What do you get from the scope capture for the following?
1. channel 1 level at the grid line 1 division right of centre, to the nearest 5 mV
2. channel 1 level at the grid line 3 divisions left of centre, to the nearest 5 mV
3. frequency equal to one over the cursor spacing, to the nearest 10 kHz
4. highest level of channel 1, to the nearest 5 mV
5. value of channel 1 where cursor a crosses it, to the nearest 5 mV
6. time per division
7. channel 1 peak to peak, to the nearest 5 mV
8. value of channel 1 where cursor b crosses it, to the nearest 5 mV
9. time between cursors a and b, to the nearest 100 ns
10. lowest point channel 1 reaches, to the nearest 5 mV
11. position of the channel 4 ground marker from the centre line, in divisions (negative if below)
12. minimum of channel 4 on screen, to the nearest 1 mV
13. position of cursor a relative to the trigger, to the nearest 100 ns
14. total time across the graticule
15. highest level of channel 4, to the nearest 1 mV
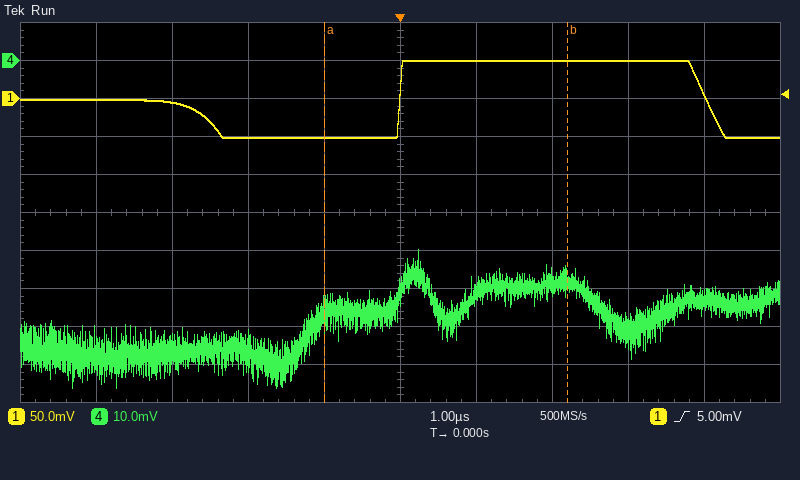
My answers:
50 mV
-5 mV
310 kHz
50 mV
-50 mV
1 µs
100 mV
50 mV
3.2 µs
-50 mV
+4.0 div
-86 mV
-1.0 µs
10 µs
-50 mV
